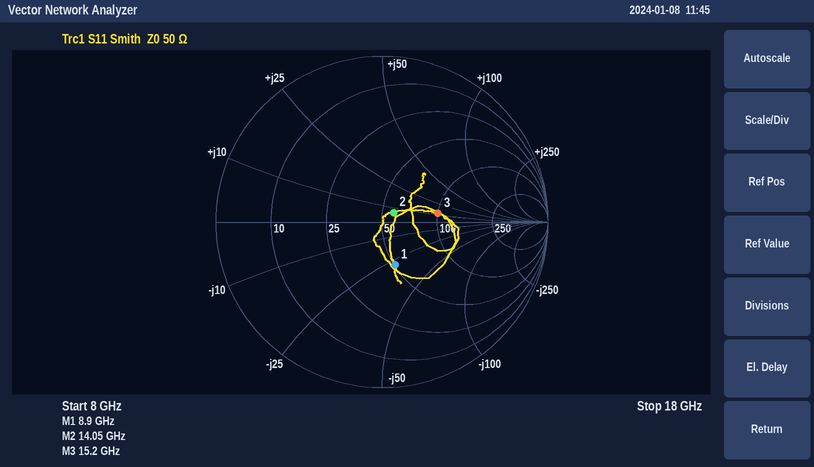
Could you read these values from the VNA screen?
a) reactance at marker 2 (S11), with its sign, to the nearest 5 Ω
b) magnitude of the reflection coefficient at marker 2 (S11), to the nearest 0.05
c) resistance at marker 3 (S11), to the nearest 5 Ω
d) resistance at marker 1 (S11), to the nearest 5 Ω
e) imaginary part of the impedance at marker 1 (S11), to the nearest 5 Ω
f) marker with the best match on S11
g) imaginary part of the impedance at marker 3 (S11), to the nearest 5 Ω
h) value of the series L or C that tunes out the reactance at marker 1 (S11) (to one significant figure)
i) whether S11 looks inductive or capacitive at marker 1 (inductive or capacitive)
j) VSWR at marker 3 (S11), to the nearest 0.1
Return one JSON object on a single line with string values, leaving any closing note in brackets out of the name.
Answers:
{"reactance at marker 2 (S11), with its sign, to the nearest 5 Ω": "+5 Ω", "magnitude of the reflection coefficient at marker 2 (S11), to the nearest 0.05": "0.10", "resistance at marker 3 (S11), to the nearest 5 Ω": "100 Ω", "resistance at marker 1 (S11), to the nearest 5 Ω": "50 Ω", "imaginary part of the impedance at marker 1 (S11), to the nearest 5 Ω": "-30 Ω", "marker with the best match on S11": "marker 2", "imaginary part of the impedance at marker 3 (S11), to the nearest 5 Ω": "+10 Ω", "value of the series L or C that tunes out the reactance at marker 1 (S11)": "500 pH", "whether S11 looks inductive or capacitive at marker 1": "capacitive", "VSWR at marker 3 (S11), to the nearest 0.1": "2.0"}
